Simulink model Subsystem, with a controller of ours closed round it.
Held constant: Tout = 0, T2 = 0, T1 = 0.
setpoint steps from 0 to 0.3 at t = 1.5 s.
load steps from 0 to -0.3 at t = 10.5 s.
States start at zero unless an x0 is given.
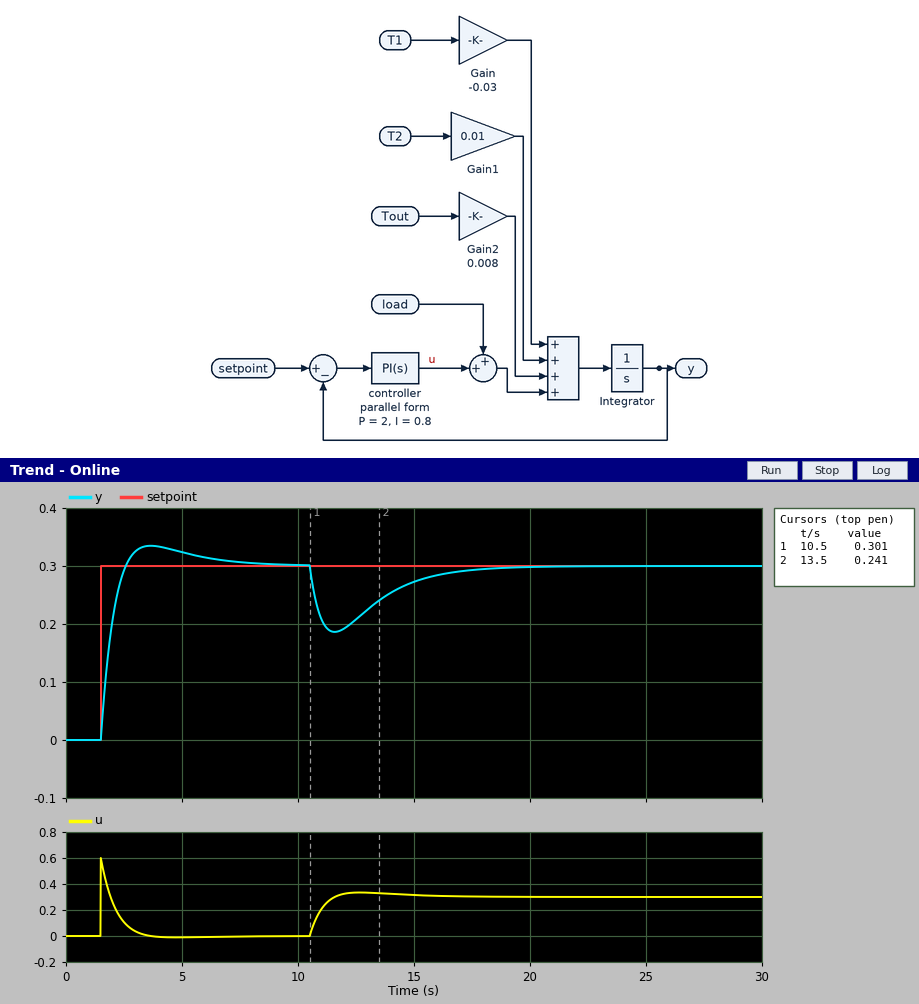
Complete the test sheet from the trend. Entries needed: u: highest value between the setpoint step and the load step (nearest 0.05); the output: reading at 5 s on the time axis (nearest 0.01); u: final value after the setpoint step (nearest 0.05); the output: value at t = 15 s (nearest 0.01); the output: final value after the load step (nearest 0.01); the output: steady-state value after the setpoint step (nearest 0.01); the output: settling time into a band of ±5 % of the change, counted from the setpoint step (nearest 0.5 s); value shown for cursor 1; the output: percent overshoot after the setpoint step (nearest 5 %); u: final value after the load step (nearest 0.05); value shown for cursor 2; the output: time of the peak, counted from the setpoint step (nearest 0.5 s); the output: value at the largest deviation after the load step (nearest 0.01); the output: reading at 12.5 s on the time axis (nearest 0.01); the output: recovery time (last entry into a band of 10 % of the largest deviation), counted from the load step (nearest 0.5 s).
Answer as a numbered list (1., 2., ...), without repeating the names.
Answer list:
1. 0.60
2. 0.32
3. 0.00
4. 0.27
5. 0.30
6. 0.30
7. 4.5 s
8. 0.301
9. 10 %
10. 0.30
11. 0.241
12. 2.0 s
13. 0.19
14. 0.21
15. 6.0 s
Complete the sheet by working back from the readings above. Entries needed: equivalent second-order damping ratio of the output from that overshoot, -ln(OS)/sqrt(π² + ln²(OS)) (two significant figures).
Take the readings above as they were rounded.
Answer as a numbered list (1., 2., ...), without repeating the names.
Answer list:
1. 0.59
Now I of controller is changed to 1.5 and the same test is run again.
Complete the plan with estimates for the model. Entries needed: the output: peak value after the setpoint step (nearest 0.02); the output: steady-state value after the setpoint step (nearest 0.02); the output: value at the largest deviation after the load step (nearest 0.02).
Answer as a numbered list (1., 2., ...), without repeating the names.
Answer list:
1. 0.36
2. 0.30
3. 0.20
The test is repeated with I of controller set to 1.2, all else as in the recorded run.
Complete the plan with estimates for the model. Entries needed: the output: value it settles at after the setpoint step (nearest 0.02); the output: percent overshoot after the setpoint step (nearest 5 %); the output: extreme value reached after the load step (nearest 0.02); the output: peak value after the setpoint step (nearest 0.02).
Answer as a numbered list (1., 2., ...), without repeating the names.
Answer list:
1. 0.30
2. 15 %
3. 0.20
4. 0.34
